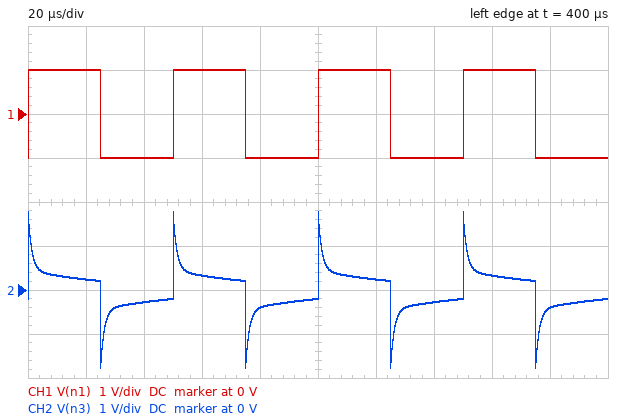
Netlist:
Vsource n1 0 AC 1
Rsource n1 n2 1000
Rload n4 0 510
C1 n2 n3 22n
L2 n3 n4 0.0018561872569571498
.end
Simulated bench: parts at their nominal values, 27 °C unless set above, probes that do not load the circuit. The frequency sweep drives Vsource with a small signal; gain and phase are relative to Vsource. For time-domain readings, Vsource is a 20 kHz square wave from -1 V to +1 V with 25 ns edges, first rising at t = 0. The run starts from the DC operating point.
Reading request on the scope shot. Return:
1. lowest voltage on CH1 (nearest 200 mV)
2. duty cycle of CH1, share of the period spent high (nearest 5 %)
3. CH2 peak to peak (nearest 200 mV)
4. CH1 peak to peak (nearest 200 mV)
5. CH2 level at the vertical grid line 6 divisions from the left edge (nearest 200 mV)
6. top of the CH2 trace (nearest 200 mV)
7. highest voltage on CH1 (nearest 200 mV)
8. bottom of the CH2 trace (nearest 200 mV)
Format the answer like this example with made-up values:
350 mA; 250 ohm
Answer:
-1.0 V; 50 %; 3.6 V; 2.0 V; 200 mV; 1.8 V; 1.0 V; -1.8 V
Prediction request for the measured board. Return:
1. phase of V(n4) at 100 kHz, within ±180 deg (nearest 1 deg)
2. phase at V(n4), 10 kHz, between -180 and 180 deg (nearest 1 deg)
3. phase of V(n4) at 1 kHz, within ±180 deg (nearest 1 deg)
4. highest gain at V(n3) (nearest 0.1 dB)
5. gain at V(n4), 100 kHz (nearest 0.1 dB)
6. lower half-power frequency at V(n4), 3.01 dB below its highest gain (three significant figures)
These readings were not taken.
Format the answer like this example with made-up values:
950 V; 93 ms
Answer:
-36 deg; 22 deg; 78 deg; 0 dB; -11.3 dB; 4.63 kHz
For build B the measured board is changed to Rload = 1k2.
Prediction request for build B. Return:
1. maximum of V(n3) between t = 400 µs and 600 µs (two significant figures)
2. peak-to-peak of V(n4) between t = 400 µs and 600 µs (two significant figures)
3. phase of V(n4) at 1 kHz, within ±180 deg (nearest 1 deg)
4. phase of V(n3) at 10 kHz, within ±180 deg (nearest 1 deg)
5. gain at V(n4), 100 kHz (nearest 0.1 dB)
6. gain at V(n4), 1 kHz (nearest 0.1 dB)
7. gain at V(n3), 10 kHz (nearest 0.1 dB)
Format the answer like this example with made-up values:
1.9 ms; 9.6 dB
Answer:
1.6 V; 1.3 V; 73 deg; 21 deg; -6.2 dB; -16.0 dB; -5.5 dB
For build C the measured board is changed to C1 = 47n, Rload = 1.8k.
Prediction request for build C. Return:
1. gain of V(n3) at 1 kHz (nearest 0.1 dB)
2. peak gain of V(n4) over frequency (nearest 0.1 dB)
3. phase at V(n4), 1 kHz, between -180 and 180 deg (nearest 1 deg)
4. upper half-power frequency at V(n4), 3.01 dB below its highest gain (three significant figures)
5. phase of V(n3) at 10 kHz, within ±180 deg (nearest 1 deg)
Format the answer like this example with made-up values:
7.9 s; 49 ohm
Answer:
-7.7 dB; -3.8 dB; 50 deg; 241 kHz; 8 deg
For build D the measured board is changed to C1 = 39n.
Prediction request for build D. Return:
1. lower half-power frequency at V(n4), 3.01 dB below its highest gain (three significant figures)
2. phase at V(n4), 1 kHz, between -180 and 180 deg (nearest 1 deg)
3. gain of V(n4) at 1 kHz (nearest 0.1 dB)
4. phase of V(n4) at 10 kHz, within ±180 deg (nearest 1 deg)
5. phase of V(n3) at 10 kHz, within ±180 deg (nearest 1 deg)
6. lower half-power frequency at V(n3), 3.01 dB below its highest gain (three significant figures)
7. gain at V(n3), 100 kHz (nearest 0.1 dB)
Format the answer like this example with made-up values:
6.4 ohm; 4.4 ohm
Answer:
2.65 kHz; 70 deg; -18.6 dB; 11 deg; 24 deg; 111 kHz; -3.4 dB
